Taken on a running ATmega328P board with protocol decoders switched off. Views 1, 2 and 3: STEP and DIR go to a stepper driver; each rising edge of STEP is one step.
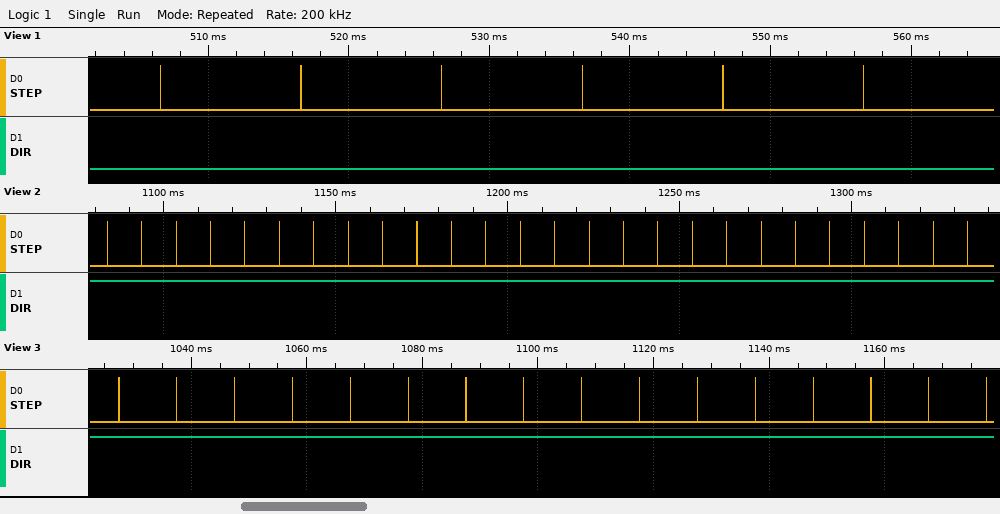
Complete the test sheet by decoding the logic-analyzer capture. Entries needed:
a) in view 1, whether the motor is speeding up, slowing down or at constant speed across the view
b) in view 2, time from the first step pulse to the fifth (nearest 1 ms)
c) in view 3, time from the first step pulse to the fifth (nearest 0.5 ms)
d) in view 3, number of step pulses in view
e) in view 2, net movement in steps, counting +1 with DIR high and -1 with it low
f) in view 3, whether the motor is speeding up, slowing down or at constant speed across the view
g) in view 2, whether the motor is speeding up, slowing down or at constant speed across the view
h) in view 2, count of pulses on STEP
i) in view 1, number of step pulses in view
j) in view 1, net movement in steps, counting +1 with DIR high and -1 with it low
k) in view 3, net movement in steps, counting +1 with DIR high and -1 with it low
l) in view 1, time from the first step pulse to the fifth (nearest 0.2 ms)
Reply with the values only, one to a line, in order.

constant speed
40 ms
40.0 ms
16
+26
constant speed
constant speed
26
6
-6
+16
40.0 ms
